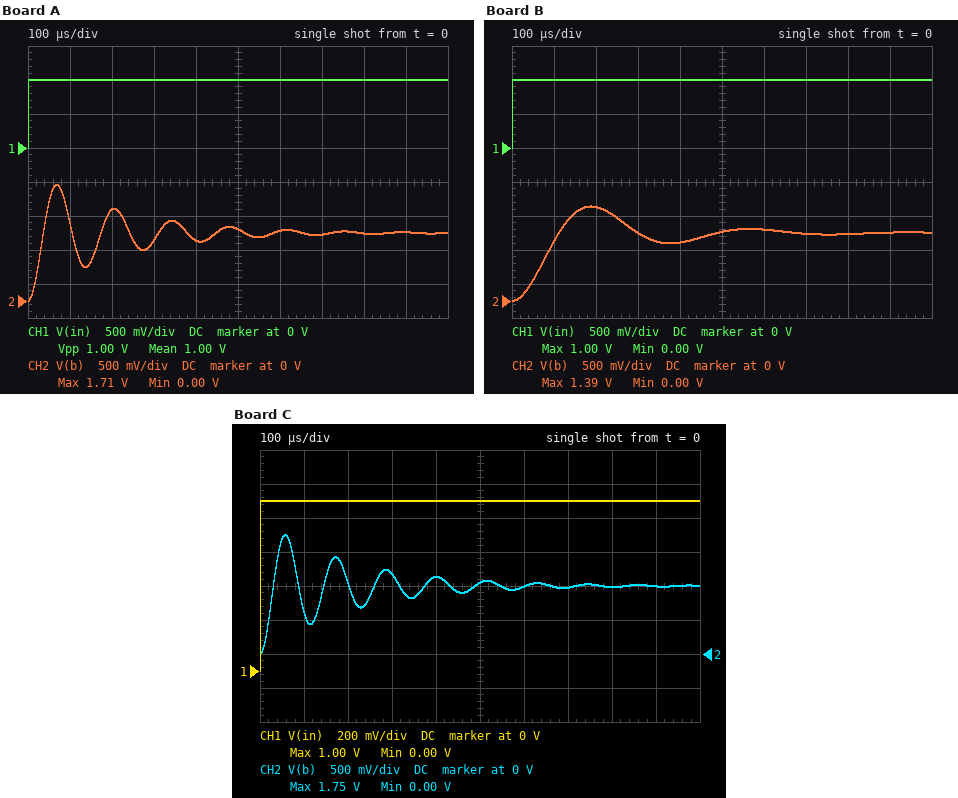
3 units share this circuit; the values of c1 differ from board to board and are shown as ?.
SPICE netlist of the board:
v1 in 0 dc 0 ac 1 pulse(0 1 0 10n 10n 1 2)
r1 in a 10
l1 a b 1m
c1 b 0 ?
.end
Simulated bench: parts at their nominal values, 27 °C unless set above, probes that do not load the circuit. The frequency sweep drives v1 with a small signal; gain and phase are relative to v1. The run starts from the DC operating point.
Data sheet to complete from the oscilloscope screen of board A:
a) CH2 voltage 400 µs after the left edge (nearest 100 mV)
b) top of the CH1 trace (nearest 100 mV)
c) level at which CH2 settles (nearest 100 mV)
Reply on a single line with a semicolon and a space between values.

900 mV; 1.0 V; 1.0 V
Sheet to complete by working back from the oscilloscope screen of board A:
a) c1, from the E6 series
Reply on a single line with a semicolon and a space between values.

470 nF
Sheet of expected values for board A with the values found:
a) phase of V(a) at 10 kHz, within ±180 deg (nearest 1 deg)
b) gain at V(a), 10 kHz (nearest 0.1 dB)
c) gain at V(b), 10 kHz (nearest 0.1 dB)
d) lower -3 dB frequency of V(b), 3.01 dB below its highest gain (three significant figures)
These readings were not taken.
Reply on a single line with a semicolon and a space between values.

19 deg; -0.5 dB; 0.9 dB; 6.40 kHz
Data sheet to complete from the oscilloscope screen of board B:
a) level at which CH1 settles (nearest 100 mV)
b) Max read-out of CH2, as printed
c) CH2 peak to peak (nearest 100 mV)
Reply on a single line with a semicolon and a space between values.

1.0 V; 1.39 V; 1.4 V
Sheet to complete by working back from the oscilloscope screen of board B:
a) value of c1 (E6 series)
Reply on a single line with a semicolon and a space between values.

3.3 µF
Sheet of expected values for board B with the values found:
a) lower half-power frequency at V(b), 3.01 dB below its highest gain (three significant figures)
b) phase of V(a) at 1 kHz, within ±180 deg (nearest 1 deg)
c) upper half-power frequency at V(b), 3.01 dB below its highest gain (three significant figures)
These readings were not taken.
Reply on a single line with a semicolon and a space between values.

1.48 kHz; -13 deg; 3.26 kHz
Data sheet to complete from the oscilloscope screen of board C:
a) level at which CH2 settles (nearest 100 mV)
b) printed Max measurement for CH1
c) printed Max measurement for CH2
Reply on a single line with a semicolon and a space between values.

1.0 V; 1.00 V; 1.75 V
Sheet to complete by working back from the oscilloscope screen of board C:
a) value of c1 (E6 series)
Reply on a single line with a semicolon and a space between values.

330 nF
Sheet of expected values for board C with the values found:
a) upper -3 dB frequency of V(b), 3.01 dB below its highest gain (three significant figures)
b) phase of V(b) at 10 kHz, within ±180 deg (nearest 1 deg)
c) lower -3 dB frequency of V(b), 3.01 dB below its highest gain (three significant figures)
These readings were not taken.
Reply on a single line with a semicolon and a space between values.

9.45 kHz; -146 deg; 7.85 kHz
